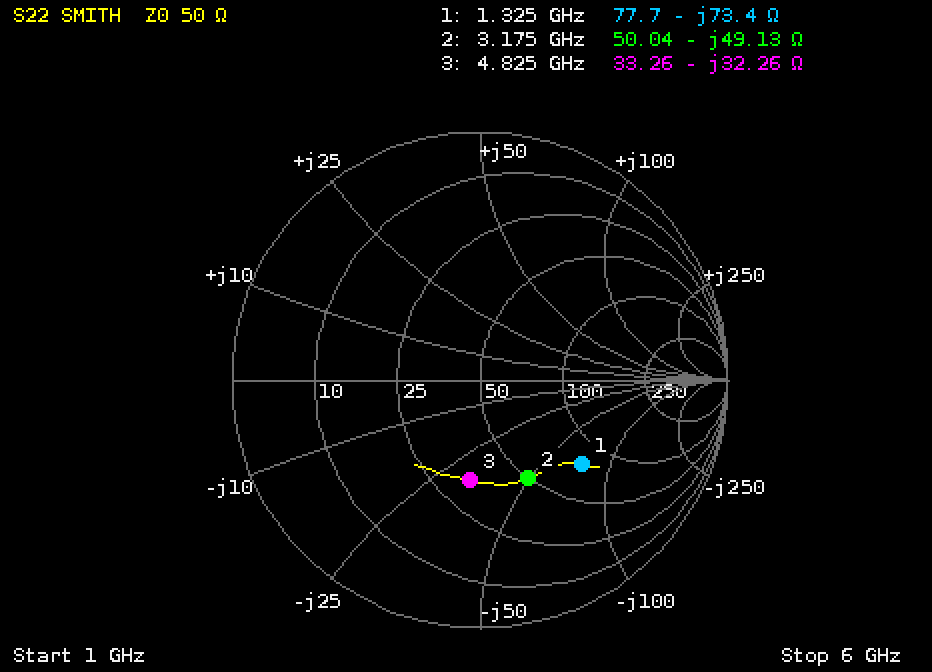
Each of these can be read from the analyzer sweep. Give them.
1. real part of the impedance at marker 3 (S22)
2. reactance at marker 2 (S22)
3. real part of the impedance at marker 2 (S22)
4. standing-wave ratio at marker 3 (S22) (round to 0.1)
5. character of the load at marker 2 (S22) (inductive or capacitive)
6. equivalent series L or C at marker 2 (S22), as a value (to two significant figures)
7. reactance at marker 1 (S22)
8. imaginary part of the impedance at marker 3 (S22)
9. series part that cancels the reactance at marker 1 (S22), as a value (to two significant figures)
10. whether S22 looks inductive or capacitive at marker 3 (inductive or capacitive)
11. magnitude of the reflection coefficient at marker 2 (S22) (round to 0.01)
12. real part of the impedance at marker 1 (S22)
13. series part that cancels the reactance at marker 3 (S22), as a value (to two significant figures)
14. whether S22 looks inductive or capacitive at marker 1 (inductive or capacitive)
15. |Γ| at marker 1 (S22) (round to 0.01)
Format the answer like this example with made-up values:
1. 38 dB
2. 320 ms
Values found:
1. 33.26 Ω
2. -49.13 Ω
3. 50.04 Ω
4. 2.4
5. capacitive
6. 1.0 pF
7. -73.4 Ω
8. -32.26 Ω
9. 8.8 nH
10. capacitive
11. 0.44
12. 77.7 Ω
13. 1.1 nH
14. capacitive
15. 0.53
